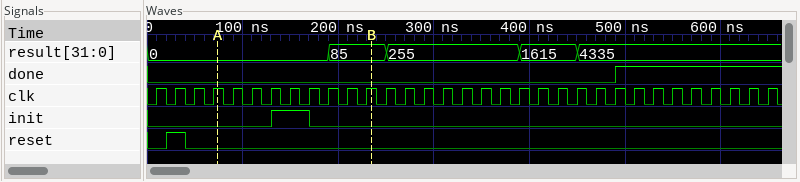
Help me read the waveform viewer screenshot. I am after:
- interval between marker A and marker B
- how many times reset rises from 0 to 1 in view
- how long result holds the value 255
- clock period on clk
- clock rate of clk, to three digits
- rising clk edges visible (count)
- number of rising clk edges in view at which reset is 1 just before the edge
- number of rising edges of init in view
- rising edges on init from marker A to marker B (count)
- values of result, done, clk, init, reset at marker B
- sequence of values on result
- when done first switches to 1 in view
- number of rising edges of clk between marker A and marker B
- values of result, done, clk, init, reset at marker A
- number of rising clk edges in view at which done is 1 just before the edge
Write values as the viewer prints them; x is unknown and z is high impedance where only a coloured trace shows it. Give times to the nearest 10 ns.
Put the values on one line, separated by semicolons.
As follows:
160 ns; 1; 140 ns; 20 ns; 50.0 MHz; 33; 1; 1; 1; result=85, done=0, clk=1, init=0, reset=0; 0, 85, 255, 1615, 4335; 490 ns; 8; result=0, done=0, clk=1, init=0, reset=0; 8
